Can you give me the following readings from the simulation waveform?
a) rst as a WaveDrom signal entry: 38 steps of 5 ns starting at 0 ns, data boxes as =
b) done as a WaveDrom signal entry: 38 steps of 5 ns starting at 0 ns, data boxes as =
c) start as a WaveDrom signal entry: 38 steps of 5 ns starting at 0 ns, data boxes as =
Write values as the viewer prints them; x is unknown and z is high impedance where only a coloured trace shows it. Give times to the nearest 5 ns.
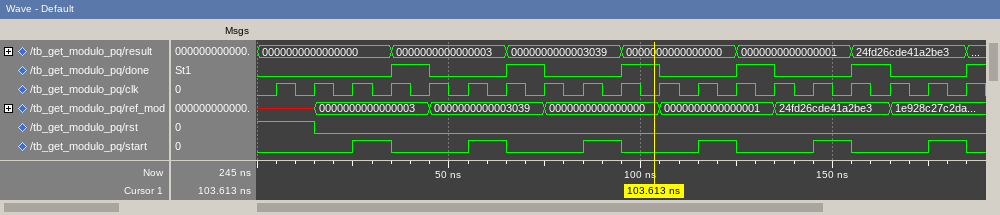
{name: 'rst', wave: '1..0..................................'}
{name: 'done', wave: '0......1.0...1.0...1.0...1.0...1.0...1'}
{name: 'start', wave: '0....1.0...1.0...1.0...1.0...1.0...1.0'}
